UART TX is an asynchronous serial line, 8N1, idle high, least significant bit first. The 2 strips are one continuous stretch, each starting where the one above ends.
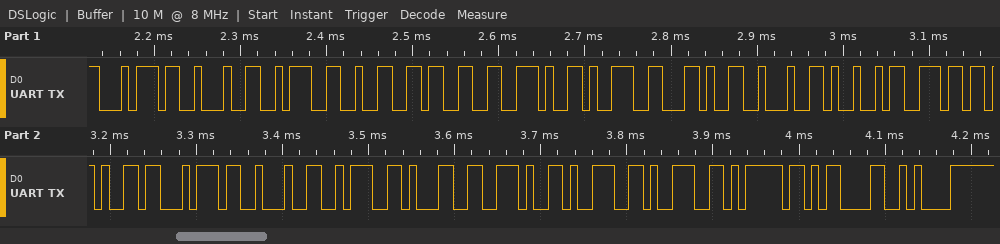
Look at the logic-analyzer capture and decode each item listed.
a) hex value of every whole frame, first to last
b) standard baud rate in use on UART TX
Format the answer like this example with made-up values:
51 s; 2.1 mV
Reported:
74 22 3A 32 33 2E 39 2C 22 49 6E 65 74 22 3A 31 2E 39 39 7D 0D 0A; 115200 baud
